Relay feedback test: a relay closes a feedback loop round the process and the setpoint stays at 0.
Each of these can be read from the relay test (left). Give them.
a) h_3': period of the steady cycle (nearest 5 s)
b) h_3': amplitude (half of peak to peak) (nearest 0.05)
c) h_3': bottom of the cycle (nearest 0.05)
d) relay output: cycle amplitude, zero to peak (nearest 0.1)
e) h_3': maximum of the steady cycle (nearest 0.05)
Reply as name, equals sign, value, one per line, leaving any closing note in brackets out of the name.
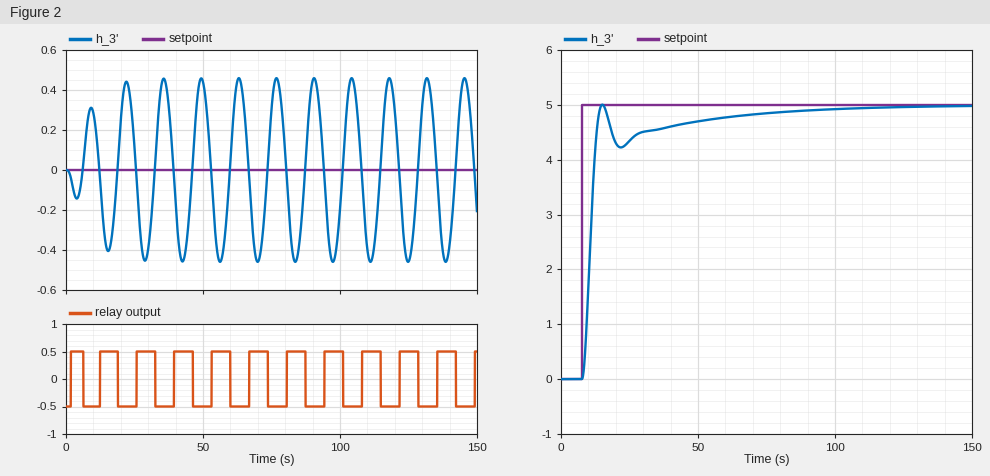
h_3': period of the steady cycle = 15 s
h_3': amplitude (half of peak to peak) = 0.45
h_3': bottom of the cycle = -0.45
relay output: cycle amplitude, zero to peak = 0.5
h_3': maximum of the steady cycle = 0.45
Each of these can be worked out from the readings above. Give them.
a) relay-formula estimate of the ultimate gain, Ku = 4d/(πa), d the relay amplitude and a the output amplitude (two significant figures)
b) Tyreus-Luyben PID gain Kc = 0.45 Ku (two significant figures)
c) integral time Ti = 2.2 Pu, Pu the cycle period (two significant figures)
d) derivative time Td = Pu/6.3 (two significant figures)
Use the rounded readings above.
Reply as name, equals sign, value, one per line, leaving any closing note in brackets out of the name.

relay-formula estimate of the ultimate gain, Ku = 4d/(πa), d the relay amplitude and a the output amplitude = 1.4
Tyreus-Luyben PID gain Kc = 0.45 Ku = 0.63
integral time Ti = 2.2 Pu, Pu the cycle period = 33 s
derivative time Td = Pu/6.3 = 2.4 s
